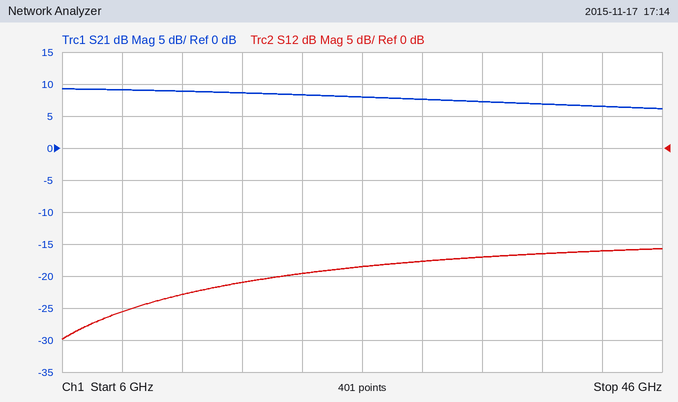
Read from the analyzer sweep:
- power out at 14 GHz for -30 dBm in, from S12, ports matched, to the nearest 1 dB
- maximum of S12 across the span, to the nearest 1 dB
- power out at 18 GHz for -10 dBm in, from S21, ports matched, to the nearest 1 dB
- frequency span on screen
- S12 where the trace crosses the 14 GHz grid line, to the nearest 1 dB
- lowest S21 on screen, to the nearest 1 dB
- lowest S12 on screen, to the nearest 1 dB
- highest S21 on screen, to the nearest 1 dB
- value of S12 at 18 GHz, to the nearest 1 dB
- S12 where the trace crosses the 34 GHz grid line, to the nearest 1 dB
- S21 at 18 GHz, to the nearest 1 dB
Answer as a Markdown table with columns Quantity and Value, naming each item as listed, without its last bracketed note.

| Quantity | Value |
|---|---|
| power out at 14 GHz for -30 dBm in, from S12, ports matched, to the nearest 1 dB | -53 dBm |
| maximum of S12 across the span, to the nearest 1 dB | -16 dB |
| power out at 18 GHz for -10 dBm in, from S21, ports matched, to the nearest 1 dB | -1 dBm |
| frequency span on screen | 40 GHz |
| S12 where the trace crosses the 14 GHz grid line, to the nearest 1 dB | -23 dB |
| lowest S21 on screen, to the nearest 1 dB | 6 dB |
| lowest S12 on screen, to the nearest 1 dB | -30 dB |
| highest S21 on screen, to the nearest 1 dB | 9 dB |
| value of S12 at 18 GHz, to the nearest 1 dB | -21 dB |
| S12 where the trace crosses the 34 GHz grid line, to the nearest 1 dB | -17 dB |
| S21 at 18 GHz, to the nearest 1 dB | 9 dB |
